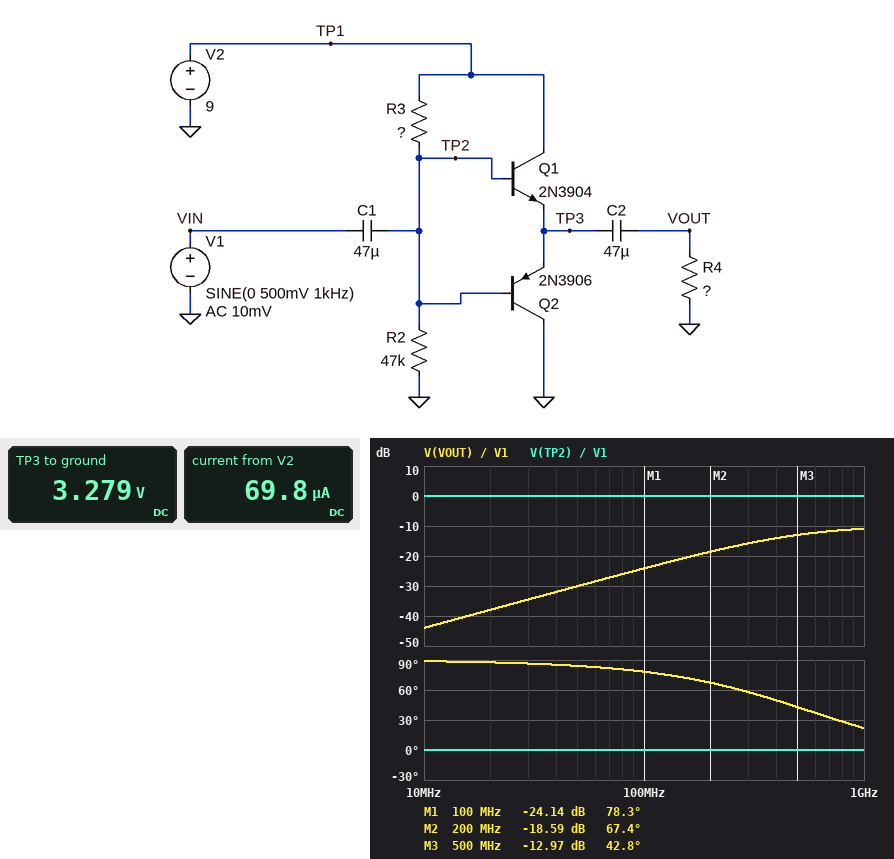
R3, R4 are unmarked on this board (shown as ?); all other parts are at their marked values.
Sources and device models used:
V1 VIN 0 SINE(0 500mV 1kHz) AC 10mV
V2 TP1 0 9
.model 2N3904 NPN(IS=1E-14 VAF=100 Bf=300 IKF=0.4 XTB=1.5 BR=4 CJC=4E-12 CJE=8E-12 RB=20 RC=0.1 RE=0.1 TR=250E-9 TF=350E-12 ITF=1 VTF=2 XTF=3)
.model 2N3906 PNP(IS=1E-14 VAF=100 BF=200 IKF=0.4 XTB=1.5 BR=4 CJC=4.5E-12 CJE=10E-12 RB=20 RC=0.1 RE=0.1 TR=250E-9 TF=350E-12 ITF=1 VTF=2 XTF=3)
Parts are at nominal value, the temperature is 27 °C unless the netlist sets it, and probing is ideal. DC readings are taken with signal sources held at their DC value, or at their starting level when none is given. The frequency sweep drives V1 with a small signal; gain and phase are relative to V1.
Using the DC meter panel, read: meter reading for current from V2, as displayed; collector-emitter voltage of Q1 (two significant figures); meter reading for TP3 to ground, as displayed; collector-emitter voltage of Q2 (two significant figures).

69.8 µA
5.7 V
3.279 V
-3.3 V
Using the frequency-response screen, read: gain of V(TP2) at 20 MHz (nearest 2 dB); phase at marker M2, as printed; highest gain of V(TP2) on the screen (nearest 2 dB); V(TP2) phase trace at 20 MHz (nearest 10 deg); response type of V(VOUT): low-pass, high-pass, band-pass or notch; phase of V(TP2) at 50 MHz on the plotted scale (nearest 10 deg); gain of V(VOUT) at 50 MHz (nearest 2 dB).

0 dB
67.4 deg
0 dB
0 deg
high-pass
0 deg
-30 dB
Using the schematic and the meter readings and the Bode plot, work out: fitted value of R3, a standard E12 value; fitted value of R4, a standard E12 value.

82 kΩ
5.6 Ω
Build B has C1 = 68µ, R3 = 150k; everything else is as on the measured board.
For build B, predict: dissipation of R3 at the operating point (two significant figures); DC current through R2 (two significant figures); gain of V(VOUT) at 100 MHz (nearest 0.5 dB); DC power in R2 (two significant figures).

310 µW
46 µA
-24.0 dB
98 µW
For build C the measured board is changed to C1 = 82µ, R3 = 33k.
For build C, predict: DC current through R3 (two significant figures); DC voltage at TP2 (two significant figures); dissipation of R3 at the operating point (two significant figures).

110 µA
5.3 V
420 µW
